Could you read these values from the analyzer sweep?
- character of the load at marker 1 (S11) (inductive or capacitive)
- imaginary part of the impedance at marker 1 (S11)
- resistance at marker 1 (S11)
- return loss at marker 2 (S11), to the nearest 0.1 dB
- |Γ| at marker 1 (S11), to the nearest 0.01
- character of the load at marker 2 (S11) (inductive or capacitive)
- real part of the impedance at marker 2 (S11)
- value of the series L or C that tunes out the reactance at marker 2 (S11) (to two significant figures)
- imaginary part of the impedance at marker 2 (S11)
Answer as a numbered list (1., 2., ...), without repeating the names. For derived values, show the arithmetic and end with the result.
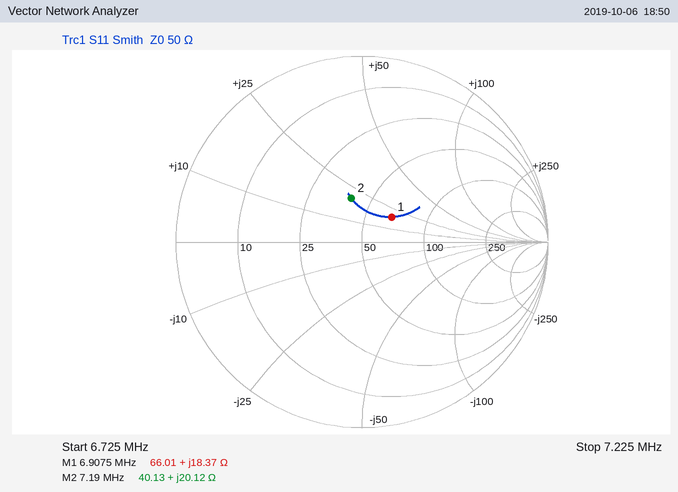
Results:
1. inductive
2. +18.37 Ω
3. 66.01 Ω
4. 12.3 dB
5. 0.21
6. inductive
7. 40.13 Ω
8. C = 1/(2π × 7.19 MHz × 20.12 Ω) ≈ 1.1 nF
9. +20.12 Ω
